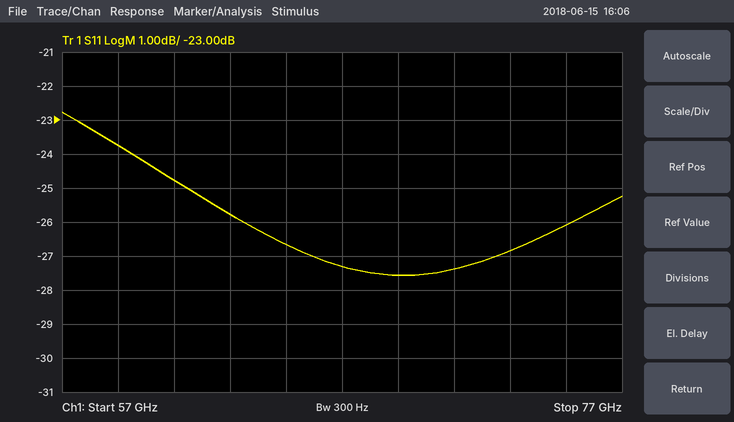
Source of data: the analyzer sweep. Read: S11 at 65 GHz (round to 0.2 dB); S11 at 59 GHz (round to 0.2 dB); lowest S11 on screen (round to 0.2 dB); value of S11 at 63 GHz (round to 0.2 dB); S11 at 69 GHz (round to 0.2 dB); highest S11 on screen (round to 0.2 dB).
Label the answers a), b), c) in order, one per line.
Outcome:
a) -26.6 dB
b) -23.8 dB
c) -27.6 dB
d) -25.8 dB
e) -27.6 dB
f) -22.8 dB
